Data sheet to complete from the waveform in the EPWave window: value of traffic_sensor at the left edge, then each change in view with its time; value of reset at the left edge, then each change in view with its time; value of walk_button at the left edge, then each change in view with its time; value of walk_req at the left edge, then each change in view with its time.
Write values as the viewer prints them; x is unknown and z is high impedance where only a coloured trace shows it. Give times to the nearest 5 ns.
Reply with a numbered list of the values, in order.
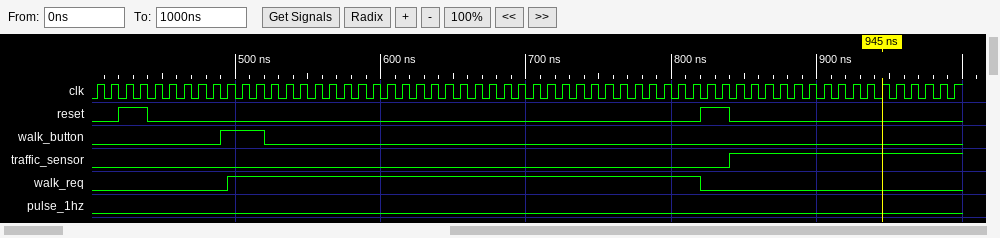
1. 0, 1 at 840 ns
2. 0, 1 at 420 ns, 0 at 440 ns, 1 at 820 ns, 0 at 840 ns
3. 0, 1 at 490 ns, 0 at 520 ns
4. 0, 1 at 495 ns, 0 at 820 ns
